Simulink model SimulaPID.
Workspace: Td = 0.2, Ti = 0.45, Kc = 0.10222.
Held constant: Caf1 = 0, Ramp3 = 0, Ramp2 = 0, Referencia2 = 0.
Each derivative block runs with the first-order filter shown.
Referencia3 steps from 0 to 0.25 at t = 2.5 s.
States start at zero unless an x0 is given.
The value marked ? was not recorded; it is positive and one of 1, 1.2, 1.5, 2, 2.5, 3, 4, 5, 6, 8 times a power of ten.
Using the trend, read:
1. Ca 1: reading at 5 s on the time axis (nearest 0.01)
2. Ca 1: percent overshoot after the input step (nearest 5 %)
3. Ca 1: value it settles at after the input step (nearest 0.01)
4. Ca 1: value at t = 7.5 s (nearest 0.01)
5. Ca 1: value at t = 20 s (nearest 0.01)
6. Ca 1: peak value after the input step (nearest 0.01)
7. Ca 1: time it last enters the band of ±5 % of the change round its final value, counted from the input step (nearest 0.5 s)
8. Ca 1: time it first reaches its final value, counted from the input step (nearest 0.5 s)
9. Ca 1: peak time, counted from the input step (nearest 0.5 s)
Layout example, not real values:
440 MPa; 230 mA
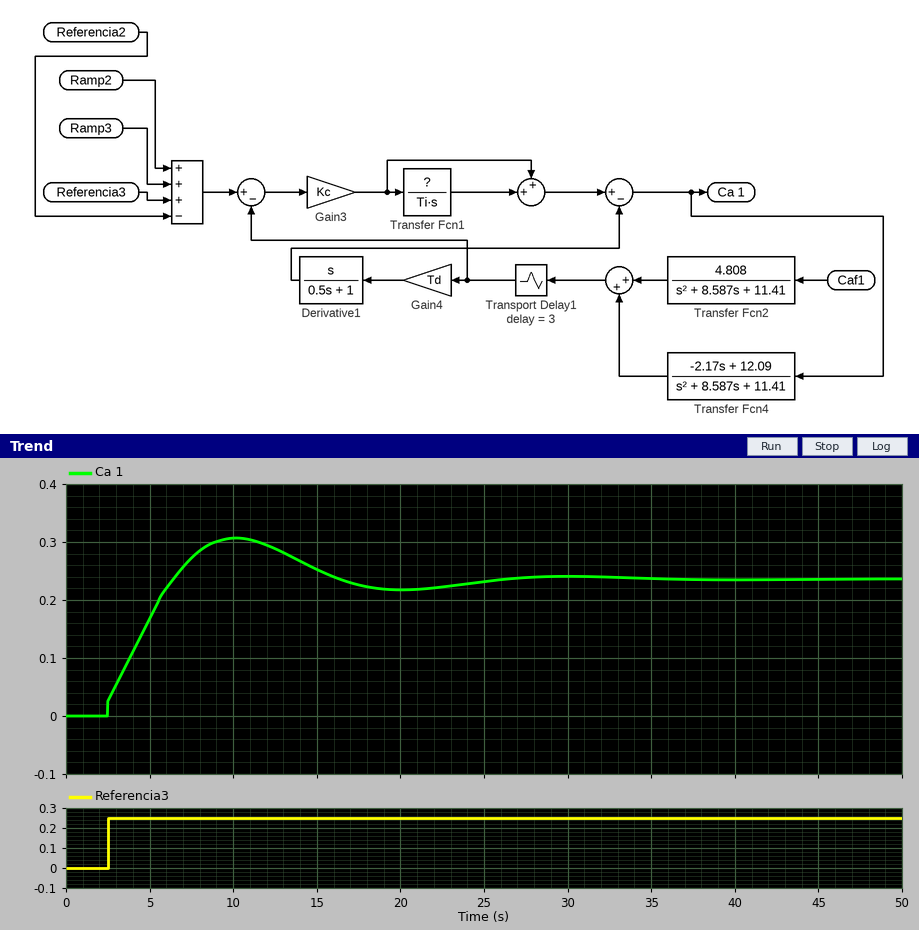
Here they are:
0.17; 30 %; 0.24; 0.27; 0.22; 0.31; 20.5 s; 4.0 s; 7.5 s
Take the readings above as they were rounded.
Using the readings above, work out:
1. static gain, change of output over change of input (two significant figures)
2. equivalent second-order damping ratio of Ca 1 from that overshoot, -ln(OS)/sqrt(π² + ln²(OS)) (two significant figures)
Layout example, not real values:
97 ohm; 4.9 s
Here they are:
0.96; 0.36
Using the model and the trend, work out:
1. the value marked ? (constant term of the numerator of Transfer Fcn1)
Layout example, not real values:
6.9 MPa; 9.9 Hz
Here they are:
1
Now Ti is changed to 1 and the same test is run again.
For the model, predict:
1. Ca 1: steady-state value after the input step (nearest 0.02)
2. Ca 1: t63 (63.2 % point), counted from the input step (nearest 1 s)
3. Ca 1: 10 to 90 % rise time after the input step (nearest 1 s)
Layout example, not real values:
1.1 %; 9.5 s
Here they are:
0.24; 6 s; 12 s
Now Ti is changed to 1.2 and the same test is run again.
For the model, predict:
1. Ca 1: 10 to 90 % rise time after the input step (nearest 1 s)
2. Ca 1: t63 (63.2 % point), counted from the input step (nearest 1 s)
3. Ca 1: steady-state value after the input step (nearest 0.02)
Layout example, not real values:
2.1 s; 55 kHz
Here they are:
17 s; 7 s; 0.24
